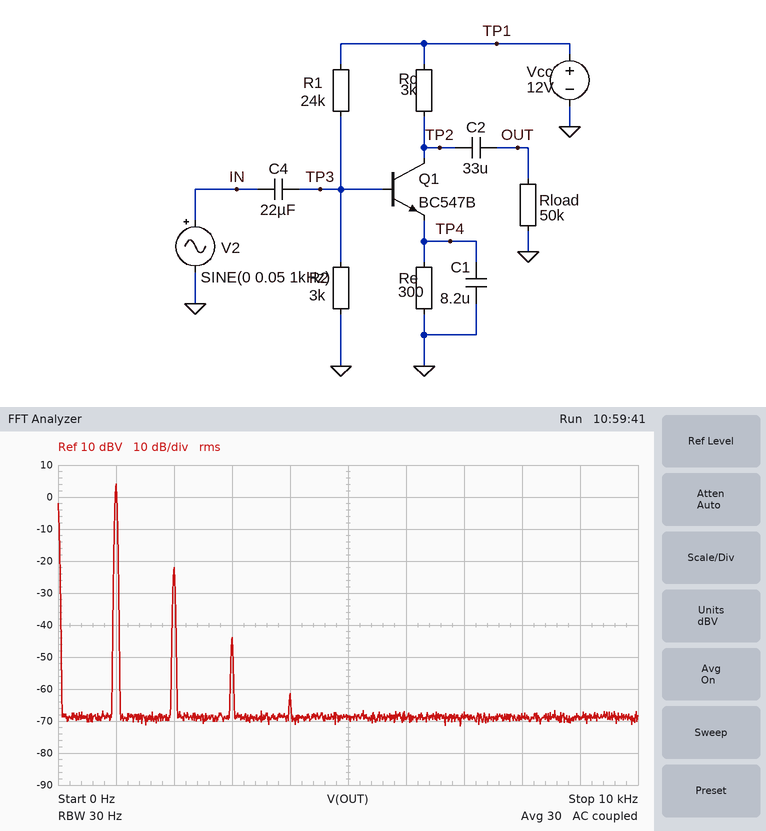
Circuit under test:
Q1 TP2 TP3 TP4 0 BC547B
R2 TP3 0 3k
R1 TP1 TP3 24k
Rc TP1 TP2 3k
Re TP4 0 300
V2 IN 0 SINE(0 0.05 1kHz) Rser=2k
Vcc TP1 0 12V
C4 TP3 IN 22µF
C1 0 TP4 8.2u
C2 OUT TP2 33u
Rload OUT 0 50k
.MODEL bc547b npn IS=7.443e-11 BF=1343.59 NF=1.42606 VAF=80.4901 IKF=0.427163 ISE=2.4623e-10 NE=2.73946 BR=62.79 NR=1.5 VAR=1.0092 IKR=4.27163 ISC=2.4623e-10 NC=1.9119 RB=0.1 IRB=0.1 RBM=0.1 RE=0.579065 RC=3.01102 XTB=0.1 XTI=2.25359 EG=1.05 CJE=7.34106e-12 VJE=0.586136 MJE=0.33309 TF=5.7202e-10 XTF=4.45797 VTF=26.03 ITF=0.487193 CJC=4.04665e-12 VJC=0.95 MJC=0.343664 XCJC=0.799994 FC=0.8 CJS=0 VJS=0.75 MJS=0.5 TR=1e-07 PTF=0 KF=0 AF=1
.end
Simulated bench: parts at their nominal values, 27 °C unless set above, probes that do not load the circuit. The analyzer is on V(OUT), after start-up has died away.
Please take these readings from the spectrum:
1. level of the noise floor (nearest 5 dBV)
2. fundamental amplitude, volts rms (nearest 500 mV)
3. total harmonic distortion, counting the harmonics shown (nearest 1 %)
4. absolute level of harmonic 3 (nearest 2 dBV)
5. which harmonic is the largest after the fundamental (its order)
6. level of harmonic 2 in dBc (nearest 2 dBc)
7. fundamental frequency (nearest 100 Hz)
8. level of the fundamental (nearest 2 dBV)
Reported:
-70 dBV
1.5 V
5 %
-44 dBV
2
-26 dBc
1.0 kHz
4 dBV
